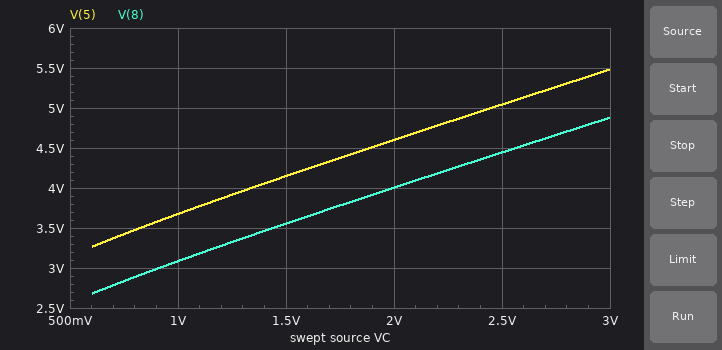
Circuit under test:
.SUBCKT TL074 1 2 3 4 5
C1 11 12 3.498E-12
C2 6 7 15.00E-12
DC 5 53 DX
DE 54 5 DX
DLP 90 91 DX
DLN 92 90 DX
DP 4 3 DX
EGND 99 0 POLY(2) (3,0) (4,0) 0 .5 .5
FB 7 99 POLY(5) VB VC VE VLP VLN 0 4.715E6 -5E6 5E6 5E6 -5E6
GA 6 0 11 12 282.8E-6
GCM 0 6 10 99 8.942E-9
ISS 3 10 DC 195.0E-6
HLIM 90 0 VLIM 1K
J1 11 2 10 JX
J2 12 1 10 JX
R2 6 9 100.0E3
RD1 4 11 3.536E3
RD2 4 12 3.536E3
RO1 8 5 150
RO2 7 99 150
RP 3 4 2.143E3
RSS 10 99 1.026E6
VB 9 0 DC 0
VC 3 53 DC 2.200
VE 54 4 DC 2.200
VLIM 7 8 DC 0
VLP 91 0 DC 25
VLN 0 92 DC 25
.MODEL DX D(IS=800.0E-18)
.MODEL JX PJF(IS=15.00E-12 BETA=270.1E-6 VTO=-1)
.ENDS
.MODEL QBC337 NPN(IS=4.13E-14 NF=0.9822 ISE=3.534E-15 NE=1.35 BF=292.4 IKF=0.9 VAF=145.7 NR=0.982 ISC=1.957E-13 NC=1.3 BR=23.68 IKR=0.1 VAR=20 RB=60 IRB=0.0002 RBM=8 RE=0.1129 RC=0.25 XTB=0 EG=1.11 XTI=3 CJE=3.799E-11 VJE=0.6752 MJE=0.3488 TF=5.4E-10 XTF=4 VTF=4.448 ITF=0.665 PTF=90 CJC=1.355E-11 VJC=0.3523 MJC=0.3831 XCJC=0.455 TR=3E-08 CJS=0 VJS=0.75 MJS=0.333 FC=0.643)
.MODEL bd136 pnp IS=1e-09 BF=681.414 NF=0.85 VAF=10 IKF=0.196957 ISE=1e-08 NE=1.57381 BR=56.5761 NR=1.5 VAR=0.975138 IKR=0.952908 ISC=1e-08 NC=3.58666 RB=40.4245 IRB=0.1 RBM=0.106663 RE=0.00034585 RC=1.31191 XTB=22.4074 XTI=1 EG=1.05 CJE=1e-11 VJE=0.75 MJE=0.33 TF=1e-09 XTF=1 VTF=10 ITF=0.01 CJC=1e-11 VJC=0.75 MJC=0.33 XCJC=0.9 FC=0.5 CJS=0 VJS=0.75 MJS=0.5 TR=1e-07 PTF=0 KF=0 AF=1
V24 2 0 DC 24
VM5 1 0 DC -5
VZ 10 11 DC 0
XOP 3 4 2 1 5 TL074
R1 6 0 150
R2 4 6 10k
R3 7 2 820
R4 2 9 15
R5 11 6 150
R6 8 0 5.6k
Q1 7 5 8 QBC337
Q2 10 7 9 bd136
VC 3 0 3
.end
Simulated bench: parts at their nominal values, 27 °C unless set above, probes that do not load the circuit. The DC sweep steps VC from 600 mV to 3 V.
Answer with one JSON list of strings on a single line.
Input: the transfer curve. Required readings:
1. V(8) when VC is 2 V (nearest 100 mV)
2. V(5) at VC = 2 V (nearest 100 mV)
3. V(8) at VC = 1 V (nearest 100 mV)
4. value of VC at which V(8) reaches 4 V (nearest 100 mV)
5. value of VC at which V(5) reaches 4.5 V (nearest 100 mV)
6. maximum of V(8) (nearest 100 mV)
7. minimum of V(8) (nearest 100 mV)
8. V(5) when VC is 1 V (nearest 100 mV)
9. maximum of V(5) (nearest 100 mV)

["4.0 V", "4.6 V", "3.1 V", "2.0 V", "1.9 V", "4.9 V", "2.7 V", "3.7 V", "5.5 V"]
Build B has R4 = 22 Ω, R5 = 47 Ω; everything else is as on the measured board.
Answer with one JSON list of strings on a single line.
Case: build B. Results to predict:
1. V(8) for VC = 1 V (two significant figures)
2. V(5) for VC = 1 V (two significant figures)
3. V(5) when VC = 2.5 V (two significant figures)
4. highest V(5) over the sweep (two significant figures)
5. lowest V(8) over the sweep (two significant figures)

["3.4 V", "4.0 V", "5.8 V", "6.4 V", "2.9 V"]
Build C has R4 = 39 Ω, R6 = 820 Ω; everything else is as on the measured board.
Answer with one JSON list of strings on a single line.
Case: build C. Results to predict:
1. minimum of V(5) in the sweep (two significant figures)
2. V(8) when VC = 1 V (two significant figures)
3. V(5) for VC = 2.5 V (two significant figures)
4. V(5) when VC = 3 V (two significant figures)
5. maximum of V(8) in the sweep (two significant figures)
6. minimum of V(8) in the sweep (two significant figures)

["1.1 V", "610 mV", "1.7 V", "1.8 V", "1.2 V", "490 mV"]
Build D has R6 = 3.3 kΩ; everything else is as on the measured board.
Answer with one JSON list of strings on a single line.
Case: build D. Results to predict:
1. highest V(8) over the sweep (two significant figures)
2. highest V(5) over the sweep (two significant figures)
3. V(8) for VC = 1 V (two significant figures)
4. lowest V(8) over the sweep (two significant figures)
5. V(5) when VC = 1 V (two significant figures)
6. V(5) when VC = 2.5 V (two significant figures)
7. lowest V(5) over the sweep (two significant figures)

["2.9 V", "3.5 V", "1.8 V", "1.6 V", "2.4 V", "3.2 V", "2.2 V"]
